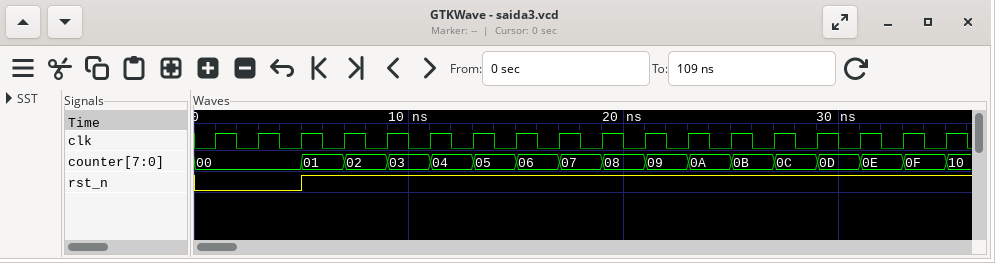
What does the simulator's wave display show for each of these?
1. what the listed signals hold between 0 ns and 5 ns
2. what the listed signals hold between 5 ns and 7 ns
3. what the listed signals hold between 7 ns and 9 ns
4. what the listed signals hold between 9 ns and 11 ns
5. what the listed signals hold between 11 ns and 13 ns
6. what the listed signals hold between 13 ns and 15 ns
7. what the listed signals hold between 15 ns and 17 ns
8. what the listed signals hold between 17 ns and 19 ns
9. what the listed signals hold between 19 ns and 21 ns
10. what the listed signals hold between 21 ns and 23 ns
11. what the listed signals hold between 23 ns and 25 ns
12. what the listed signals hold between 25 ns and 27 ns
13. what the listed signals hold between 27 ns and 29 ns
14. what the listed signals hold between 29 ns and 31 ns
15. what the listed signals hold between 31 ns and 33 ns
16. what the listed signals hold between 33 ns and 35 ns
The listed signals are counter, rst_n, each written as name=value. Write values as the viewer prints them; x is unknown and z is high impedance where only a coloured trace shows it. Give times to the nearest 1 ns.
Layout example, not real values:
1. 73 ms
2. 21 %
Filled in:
1. counter=00, rst_n=0
2. counter=01, rst_n=1
3. counter=02, rst_n=1
4. counter=03, rst_n=1
5. counter=04, rst_n=1
6. counter=05, rst_n=1
7. counter=06, rst_n=1
8. counter=07, rst_n=1
9. counter=08, rst_n=1
10. counter=09, rst_n=1
11. counter=0A, rst_n=1
12. counter=0B, rst_n=1
13. counter=0C, rst_n=1
14. counter=0D, rst_n=1
15. counter=0E, rst_n=1
16. counter=0F, rst_n=1
